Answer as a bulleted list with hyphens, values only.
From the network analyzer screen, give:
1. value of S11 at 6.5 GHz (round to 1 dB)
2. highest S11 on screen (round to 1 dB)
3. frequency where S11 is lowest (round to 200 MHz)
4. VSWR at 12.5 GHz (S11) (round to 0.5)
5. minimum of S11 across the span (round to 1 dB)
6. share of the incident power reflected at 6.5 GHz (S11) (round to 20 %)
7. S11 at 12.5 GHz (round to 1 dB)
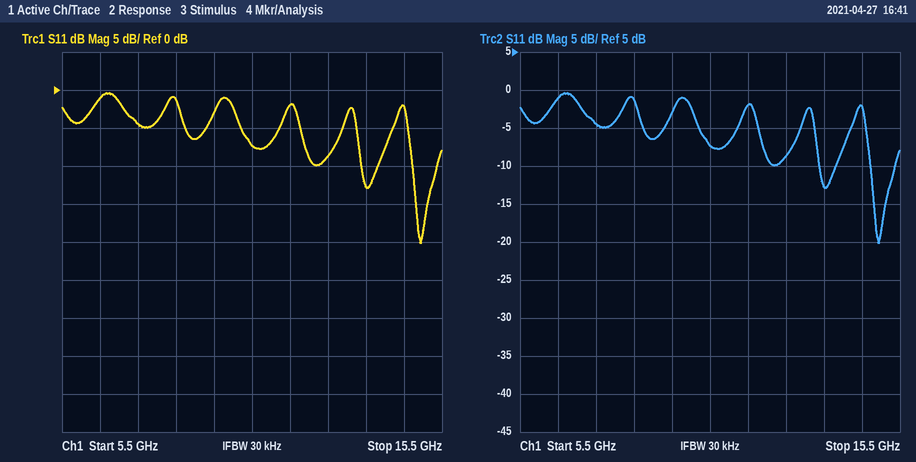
- -1 dB
- 0 dB
- 15.0 GHz
- 2.0
- -20 dB
- 80 %
- -9 dB
